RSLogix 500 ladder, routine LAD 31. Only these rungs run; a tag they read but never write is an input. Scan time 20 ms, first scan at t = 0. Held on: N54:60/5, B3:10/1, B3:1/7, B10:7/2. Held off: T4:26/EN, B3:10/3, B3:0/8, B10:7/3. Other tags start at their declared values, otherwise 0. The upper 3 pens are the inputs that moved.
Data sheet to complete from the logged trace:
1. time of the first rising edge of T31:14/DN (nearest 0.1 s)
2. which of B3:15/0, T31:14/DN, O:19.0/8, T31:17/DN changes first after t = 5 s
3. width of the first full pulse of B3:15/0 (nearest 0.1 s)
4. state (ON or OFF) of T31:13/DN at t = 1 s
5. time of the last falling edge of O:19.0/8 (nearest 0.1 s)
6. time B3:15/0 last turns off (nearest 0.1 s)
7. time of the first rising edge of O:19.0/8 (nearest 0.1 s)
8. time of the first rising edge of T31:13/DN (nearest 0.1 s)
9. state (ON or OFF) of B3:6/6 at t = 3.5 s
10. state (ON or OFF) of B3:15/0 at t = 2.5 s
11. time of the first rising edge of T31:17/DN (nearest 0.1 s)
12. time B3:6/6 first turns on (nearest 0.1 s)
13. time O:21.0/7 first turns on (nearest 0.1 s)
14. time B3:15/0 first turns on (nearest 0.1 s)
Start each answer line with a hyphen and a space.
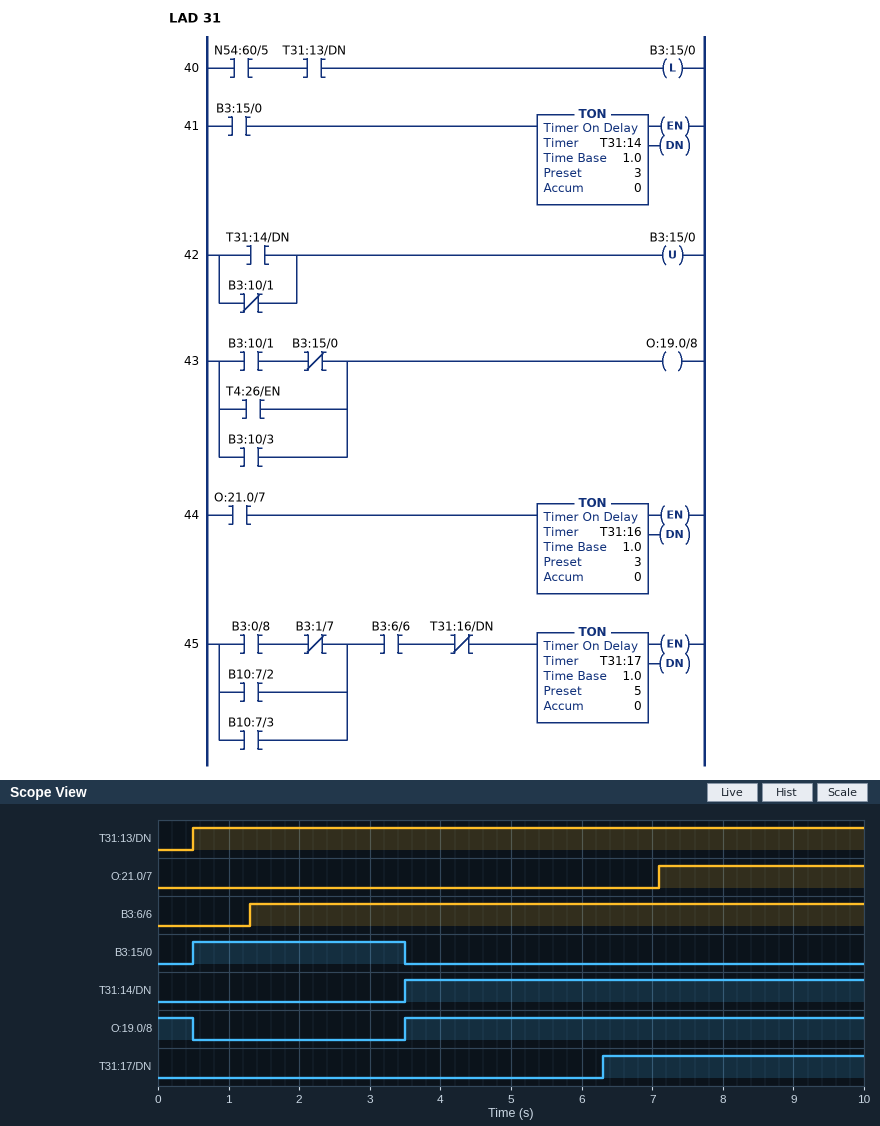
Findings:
- 3.5 s
- T31:17/DN
- 3.0 s
- ON
- 0.5 s
- 3.5 s
- 3.5 s
- 0.5 s
- ON
- ON
- 6.3 s
- 1.3 s
- 7.1 s
- 0.5 s
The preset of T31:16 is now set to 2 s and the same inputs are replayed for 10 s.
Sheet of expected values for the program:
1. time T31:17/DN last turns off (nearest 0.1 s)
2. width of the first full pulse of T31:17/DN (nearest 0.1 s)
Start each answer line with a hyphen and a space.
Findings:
- 9.1 s
- 2.8 s
